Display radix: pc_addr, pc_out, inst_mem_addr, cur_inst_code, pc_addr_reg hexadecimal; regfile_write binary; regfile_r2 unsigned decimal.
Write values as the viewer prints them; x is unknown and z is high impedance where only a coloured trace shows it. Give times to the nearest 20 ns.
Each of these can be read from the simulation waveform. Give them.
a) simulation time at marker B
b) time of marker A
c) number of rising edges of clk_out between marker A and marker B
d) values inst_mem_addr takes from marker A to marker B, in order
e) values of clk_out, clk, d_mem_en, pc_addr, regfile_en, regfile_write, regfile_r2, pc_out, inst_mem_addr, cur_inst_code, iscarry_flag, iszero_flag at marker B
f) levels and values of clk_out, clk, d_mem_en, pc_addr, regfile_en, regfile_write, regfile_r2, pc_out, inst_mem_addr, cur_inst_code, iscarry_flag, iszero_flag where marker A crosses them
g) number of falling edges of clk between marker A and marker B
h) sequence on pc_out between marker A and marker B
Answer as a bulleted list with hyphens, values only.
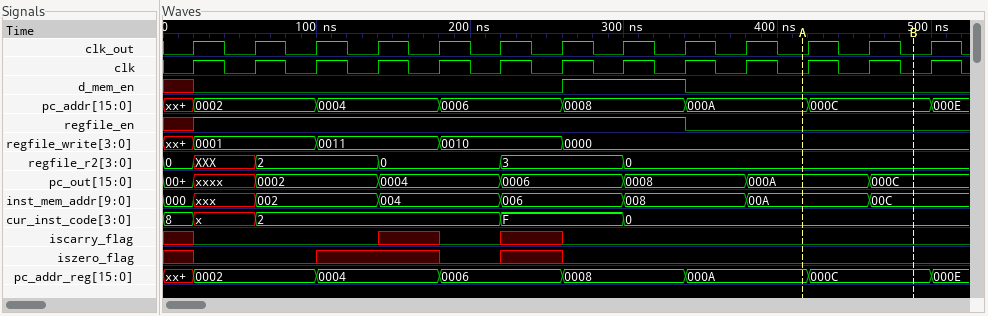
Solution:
- 480 ns
- 420 ns
- 2
- 00A, 00C
- clk_out=0, clk=0, d_mem_en=0, pc_addr=000C, regfile_en=0, regfile_write=0000, regfile_r2=0, pc_out=000C, inst_mem_addr=00C, cur_inst_code=0, iscarry_flag=0, iszero_flag=0
- clk_out=0, clk=0, d_mem_en=0, pc_addr=000A, regfile_en=0, regfile_write=0000, regfile_r2=0, pc_out=000A, inst_mem_addr=00A, cur_inst_code=0, iscarry_flag=0, iszero_flag=0
- 2
- 000A, 000C
